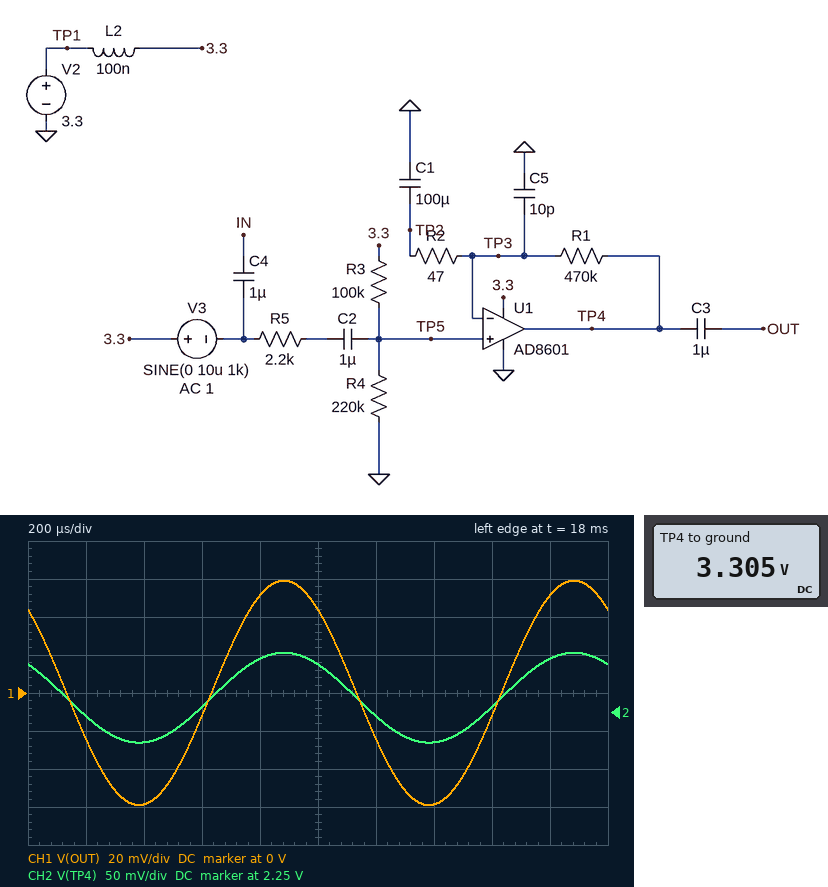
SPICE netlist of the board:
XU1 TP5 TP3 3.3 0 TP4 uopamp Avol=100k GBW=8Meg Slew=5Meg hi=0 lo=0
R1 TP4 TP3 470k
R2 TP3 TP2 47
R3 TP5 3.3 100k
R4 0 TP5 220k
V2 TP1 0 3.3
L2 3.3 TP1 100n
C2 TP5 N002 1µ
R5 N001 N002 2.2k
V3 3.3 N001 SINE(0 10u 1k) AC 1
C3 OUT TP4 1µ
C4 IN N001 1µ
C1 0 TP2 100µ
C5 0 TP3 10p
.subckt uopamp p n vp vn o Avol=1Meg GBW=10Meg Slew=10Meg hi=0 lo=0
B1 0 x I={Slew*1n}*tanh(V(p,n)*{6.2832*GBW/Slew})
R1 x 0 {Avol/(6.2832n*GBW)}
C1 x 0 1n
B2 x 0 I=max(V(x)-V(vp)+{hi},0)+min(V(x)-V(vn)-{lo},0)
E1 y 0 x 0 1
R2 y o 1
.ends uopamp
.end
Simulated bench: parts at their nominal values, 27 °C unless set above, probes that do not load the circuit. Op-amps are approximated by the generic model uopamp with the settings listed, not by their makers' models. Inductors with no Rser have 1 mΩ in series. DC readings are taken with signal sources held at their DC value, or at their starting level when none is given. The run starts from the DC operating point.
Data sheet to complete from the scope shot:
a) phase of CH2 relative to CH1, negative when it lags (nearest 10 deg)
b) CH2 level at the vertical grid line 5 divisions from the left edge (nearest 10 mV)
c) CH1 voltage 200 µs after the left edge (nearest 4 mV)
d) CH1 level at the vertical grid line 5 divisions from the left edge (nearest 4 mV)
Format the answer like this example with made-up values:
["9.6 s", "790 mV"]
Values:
["0 deg", "2.31 V", "-24 mV", "44 mV"]
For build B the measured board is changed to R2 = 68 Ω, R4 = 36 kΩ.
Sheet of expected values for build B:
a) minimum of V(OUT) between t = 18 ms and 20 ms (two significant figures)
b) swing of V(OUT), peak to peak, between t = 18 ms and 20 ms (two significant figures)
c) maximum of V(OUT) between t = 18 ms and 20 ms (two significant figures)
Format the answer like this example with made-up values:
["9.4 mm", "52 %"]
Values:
["-47 mV", "94 mV", "47 mV"]
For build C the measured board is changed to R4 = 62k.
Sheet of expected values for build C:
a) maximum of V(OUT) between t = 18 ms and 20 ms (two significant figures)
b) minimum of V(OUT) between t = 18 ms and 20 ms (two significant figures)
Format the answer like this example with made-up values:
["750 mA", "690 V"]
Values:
["58 mV", "-58 mV"]
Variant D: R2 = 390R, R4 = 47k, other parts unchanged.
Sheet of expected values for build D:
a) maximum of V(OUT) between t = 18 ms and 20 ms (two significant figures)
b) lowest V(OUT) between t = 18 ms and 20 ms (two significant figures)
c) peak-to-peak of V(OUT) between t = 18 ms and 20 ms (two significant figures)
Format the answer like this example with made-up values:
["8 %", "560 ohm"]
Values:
["11 mV", "-11 mV", "22 mV"]
